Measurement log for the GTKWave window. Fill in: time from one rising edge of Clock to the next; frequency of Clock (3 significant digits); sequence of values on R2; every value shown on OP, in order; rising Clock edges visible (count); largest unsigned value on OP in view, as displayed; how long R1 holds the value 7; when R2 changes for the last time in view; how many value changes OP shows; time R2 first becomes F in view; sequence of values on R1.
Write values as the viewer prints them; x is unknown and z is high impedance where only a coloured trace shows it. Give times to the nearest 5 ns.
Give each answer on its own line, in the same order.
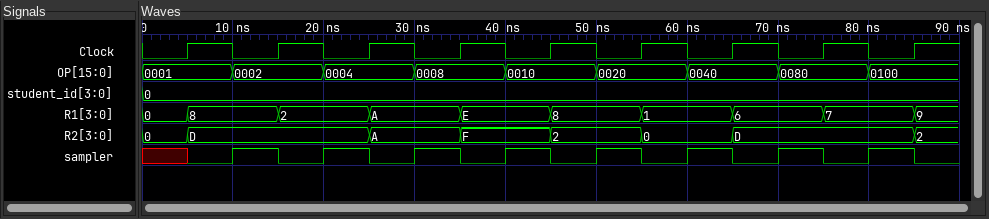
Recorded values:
10 ns
100 MHz
0, D, A, F, 2, 0, D, 2
0001, 0002, 0004, 0008, 0010, 0020, 0040, 0080, 0100
9
0100
10 ns
85 ns
8
35 ns
0, 8, 2, A, E, 8, 1, 6, 7, 9
